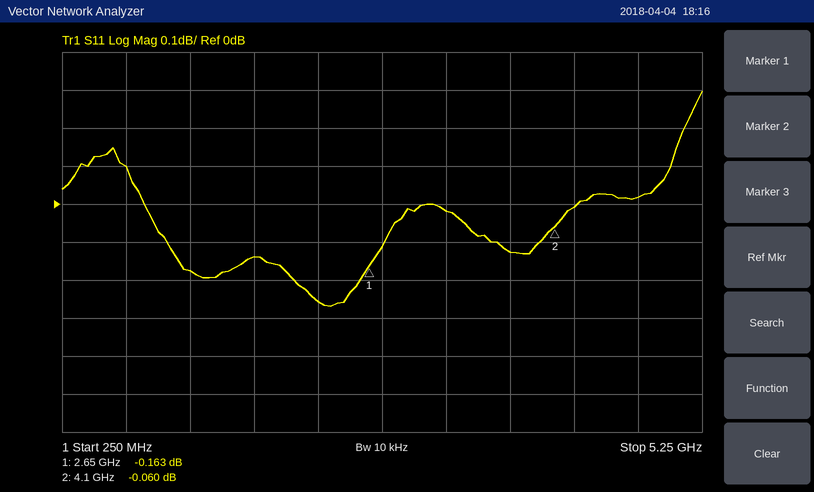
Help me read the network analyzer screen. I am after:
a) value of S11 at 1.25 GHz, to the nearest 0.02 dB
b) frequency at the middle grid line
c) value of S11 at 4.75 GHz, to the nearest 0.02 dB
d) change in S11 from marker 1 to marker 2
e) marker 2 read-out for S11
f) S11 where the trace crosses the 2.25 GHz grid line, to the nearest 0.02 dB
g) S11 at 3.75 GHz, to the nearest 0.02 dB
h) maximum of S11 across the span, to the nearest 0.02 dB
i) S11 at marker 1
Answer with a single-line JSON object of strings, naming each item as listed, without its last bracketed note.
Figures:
{"value of S11 at 1.25 GHz, to the nearest 0.02 dB": "-0.18 dB", "frequency at the middle grid line": "2.75 GHz", "value of S11 at 4.75 GHz, to the nearest 0.02 dB": "0.02 dB", "change in S11 from marker 1 to marker 2": "0.103 dB", "marker 2 read-out for S11": "-0.060 dB", "S11 where the trace crosses the 2.25 GHz grid line, to the nearest 0.02 dB": "-0.26 dB", "S11 at 3.75 GHz, to the nearest 0.02 dB": "-0.12 dB", "maximum of S11 across the span, to the nearest 0.02 dB": "0.30 dB", "S11 at marker 1": "-0.163 dB"}
